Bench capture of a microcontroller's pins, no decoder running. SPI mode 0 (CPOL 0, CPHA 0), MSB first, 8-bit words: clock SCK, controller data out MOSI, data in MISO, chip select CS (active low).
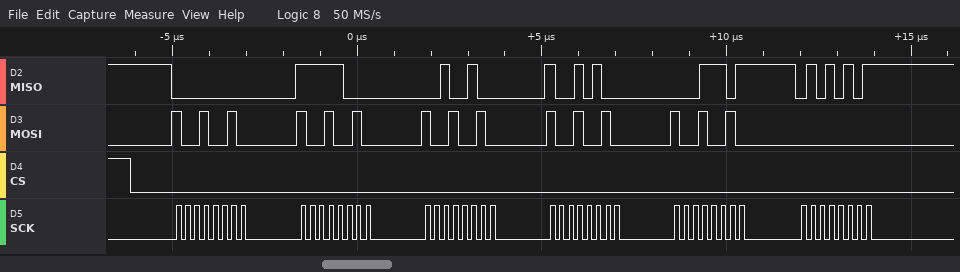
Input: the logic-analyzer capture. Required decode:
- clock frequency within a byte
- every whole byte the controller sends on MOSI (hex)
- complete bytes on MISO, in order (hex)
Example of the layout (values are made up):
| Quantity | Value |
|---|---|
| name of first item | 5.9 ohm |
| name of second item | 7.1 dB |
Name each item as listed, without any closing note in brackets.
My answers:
| Quantity | Value |
|---|---|
| clock frequency within a byte | 4 MHz |
| every whole byte the controller sends on MOSI | 0x92 0x92 0x92 0x92 0x92 0x00 |
| complete bytes on MISO, in order | 0x00 0xF8 0x24 0x94 0x1D 0x55 |
